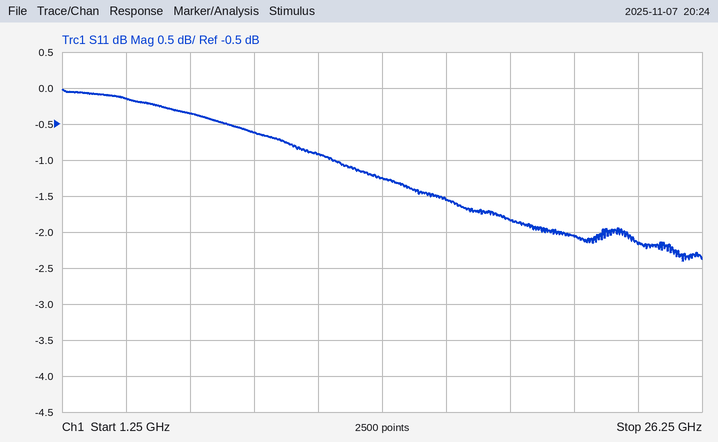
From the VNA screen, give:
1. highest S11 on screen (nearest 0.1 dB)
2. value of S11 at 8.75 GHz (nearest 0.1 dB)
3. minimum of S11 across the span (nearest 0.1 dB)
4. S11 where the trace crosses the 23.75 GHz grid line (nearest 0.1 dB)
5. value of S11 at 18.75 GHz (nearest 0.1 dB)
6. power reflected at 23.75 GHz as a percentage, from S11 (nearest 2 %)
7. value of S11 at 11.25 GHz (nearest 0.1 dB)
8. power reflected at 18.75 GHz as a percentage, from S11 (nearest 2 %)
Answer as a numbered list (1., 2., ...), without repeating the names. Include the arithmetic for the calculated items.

1. 0.0 dB
2. -0.6 dB
3. -2.4 dB
4. -2.2 dB
5. -1.8 dB
6. 10^(-2.2/10) ≈ 60 %
7. -0.9 dB
8. 10^(-1.8/10) ≈ 66 %
